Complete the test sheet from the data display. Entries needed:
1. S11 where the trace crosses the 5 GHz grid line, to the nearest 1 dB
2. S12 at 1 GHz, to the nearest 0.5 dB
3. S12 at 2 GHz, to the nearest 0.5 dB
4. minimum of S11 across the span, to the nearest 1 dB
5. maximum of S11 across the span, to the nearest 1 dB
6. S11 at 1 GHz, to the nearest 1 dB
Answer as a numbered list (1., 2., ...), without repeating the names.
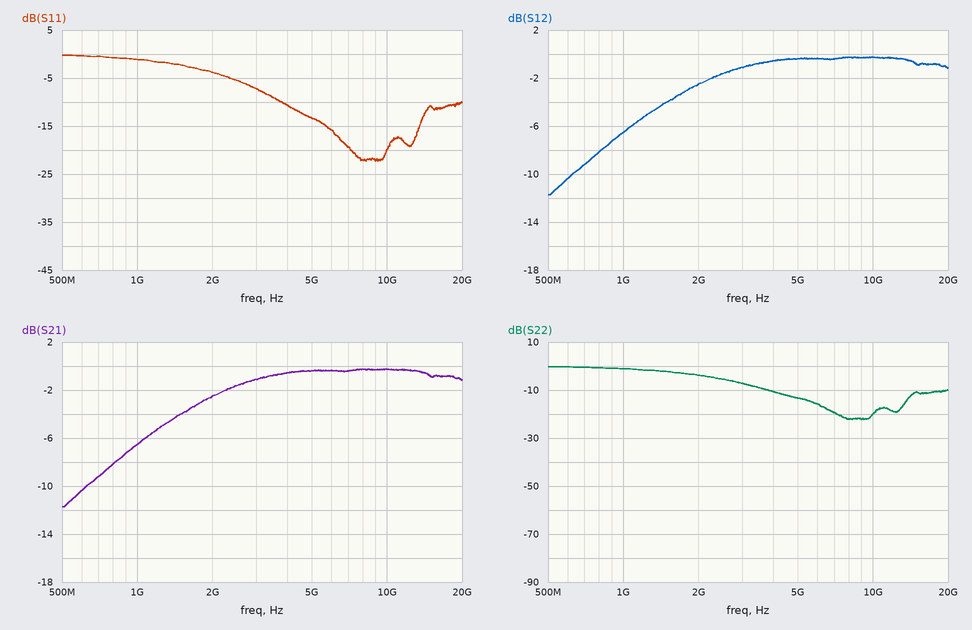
1. -13 dB
2. -6.5 dB
3. -2.5 dB
4. -22 dB
5. 0 dB
6. -1 dB
